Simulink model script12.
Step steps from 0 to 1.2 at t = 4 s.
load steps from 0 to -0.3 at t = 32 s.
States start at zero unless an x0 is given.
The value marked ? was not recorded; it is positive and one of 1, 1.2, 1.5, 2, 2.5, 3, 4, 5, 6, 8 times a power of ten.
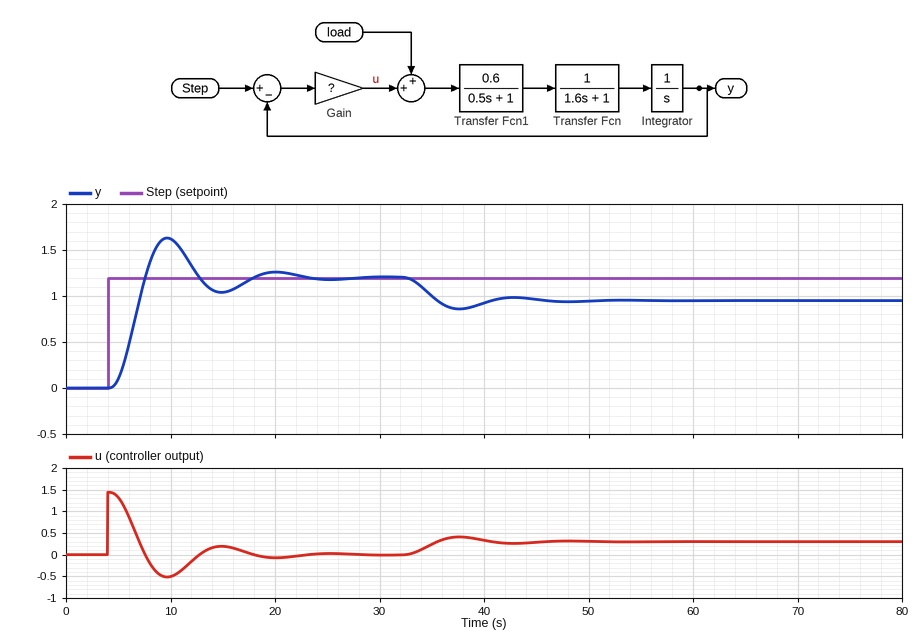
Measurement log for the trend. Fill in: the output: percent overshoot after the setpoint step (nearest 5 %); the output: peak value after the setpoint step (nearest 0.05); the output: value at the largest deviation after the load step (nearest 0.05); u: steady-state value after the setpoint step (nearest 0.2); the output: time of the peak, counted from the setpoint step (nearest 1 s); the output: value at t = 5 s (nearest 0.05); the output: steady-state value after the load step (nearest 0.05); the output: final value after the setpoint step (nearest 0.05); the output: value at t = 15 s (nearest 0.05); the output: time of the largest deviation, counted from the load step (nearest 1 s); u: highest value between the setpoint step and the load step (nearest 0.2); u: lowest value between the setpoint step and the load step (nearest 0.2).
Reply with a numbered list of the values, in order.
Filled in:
1. 35 %
2. 1.65
3. 0.85
4. 0.0
5. 6 s
6. 0.10
7. 0.95
8. 1.20
9. 1.05
10. 6 s
11. 1.4
12. -0.6
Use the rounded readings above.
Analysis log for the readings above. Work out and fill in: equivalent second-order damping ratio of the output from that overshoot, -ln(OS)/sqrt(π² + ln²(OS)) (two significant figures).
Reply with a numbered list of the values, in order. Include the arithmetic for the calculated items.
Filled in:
1. ln(0.35) = -1.050; 1.050 / sqrt(9.870 + 1.102) = 0.32
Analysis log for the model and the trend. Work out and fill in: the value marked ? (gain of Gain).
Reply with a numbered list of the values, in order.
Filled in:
1. 1.2
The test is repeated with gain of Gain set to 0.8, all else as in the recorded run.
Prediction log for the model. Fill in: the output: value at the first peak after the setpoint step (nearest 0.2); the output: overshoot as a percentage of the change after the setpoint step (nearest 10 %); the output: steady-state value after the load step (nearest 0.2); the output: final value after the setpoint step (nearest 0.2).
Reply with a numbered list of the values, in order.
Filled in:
1. 1.4
2. 20 %
3. 0.8
4. 1.2
